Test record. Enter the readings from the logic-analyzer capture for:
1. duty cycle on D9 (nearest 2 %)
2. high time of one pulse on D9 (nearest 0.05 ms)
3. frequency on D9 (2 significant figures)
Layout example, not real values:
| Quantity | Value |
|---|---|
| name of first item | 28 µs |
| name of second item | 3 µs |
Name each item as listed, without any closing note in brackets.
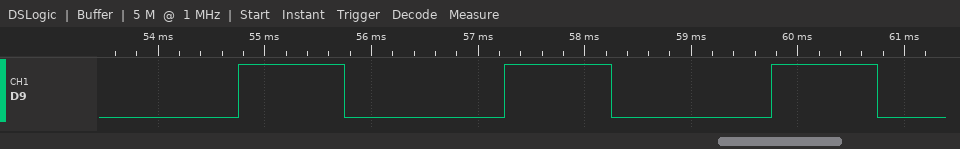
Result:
| Quantity | Value |
|---|---|
| duty cycle on D9 | 40 % |
| high time of one pulse on D9 | 1.00 ms |
| frequency on D9 | 400 Hz |
